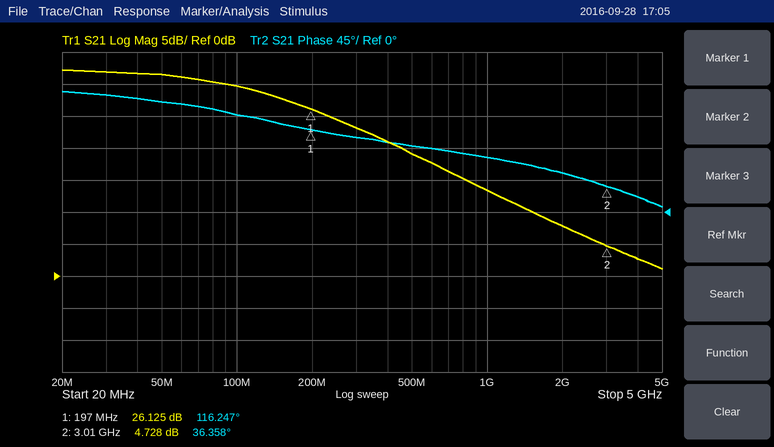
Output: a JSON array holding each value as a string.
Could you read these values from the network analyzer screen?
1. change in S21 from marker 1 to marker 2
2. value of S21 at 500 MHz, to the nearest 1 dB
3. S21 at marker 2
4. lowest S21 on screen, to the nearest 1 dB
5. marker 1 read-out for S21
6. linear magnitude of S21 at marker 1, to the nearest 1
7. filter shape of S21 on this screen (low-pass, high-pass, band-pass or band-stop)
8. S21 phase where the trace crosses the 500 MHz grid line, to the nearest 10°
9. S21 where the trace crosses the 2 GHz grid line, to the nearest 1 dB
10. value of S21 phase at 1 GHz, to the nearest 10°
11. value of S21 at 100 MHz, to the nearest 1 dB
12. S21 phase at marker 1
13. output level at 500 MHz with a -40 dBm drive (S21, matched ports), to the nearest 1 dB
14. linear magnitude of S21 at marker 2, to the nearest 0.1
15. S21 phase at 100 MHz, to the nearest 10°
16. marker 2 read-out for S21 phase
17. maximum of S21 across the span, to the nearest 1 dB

["-21.397 dB", "19 dB", "4.728 dB", "1 dB", "26.125 dB", "20", "low-pass", "90°", "8 dB", "80°", "30 dB", "116.247°", "-21 dBm", "1.7", "140°", "36.358°", "32 dB"]
